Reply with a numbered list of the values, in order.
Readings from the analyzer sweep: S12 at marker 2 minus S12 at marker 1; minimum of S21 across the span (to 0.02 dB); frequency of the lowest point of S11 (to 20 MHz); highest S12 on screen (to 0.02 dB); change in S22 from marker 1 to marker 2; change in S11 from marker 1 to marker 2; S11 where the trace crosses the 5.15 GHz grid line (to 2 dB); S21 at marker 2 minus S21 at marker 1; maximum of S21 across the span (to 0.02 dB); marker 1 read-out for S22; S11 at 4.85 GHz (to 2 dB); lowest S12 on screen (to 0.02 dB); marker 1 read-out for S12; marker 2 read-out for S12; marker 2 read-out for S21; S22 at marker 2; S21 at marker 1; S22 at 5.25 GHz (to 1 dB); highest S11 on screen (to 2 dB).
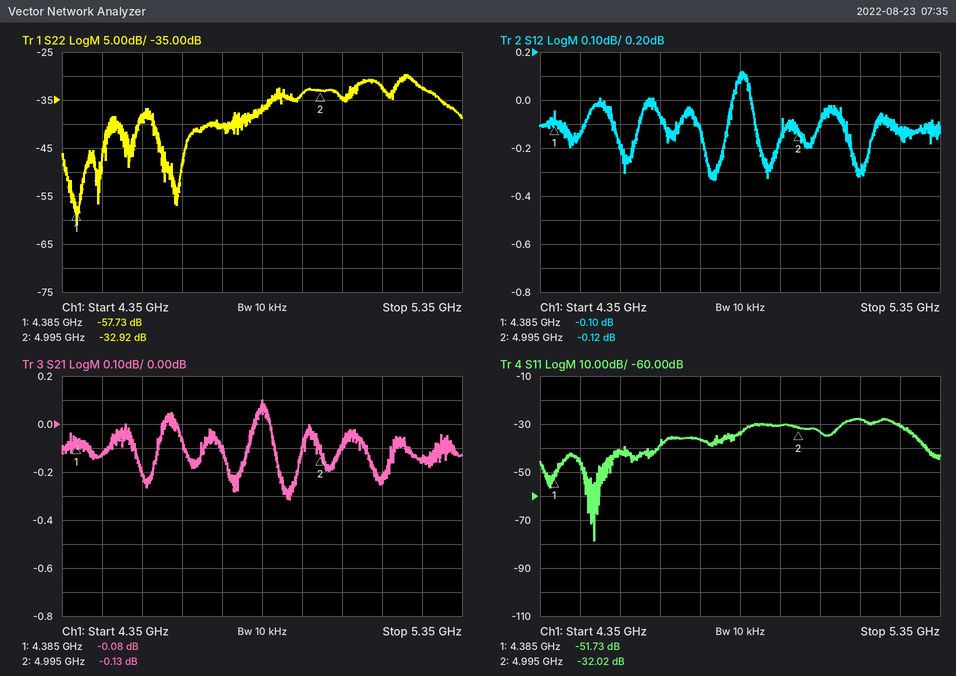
1. -0.02 dB
2. -0.32 dB
3. 4.48 GHz
4. 0.12 dB
5. 24.81 dB
6. 19.71 dB
7. -28 dB
8. -0.05 dB
9. 0.10 dB
10. -57.73 dB
11. -34 dB
12. -0.34 dB
13. -0.10 dB
14. -0.12 dB
15. -0.13 dB
16. -32.92 dB
17. -0.08 dB
18. -32 dB
19. -28 dB
